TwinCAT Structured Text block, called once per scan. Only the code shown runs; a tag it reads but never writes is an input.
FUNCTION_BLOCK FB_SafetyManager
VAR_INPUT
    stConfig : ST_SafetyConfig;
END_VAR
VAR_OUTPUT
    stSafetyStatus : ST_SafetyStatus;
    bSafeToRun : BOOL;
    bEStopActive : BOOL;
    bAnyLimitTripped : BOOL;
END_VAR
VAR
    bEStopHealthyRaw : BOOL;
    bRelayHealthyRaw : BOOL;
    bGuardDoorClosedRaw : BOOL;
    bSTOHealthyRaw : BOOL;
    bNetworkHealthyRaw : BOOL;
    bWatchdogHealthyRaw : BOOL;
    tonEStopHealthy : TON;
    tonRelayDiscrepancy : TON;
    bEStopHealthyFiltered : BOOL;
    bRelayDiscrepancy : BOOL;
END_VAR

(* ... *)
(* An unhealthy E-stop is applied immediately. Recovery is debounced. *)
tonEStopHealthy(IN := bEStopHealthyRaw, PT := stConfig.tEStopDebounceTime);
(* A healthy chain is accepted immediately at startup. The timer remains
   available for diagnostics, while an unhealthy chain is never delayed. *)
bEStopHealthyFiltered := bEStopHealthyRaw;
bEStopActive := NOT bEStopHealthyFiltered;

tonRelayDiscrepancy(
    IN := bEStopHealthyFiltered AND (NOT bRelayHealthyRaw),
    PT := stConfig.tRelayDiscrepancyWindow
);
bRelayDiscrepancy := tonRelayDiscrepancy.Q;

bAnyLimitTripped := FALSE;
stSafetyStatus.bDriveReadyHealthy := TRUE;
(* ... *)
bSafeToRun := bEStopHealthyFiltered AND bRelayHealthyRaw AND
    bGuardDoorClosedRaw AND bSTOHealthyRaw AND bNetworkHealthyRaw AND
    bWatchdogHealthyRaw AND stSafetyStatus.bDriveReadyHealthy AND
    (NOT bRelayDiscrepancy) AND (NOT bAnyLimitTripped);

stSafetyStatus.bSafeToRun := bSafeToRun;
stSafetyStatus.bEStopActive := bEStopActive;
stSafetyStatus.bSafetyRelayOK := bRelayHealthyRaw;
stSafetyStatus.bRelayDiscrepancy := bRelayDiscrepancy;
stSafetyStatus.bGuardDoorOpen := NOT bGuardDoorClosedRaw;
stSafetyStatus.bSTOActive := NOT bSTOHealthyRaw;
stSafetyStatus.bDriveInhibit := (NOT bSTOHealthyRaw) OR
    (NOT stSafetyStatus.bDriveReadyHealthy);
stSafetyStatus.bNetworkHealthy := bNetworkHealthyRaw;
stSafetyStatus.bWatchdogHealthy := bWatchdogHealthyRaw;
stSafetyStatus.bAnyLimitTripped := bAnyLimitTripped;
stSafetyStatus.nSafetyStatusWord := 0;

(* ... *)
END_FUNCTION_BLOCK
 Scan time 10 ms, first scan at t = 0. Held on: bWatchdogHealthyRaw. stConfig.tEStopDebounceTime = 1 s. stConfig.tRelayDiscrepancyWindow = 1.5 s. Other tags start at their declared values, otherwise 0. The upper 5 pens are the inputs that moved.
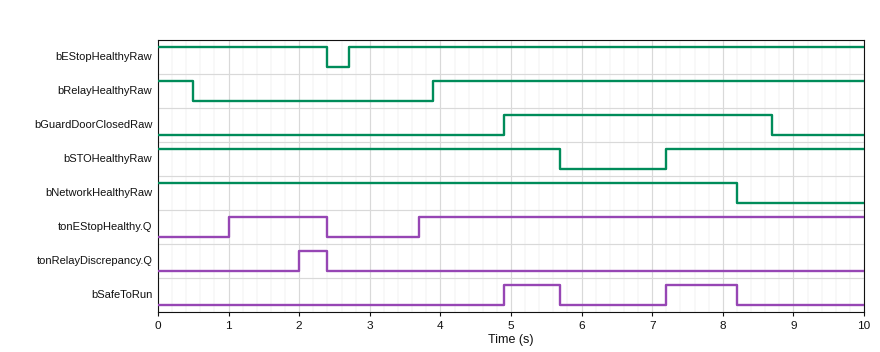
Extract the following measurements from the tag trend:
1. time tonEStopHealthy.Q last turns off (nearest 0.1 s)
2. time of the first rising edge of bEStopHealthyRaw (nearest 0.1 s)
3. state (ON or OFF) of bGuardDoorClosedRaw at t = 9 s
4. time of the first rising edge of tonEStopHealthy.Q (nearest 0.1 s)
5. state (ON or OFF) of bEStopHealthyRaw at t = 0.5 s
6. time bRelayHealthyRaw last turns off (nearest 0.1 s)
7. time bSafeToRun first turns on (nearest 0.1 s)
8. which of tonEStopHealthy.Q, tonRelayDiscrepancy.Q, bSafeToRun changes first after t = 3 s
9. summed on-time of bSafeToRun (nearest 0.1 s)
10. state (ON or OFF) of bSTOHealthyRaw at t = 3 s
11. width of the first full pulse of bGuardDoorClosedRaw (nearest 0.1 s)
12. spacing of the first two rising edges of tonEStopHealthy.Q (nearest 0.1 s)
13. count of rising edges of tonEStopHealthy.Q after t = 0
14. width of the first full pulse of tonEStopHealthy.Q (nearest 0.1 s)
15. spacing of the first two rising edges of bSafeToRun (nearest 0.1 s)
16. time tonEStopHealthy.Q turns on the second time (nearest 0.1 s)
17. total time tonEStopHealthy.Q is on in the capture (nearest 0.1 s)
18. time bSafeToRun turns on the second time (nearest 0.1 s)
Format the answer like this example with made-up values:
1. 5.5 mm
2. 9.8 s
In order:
1. 2.4 s
2. 2.7 s
3. OFF
4. 1.0 s
5. ON
6. 0.5 s
7. 4.9 s
8. tonEStopHealthy.Q
9. 1.8 s
10. ON
11. 3.8 s
12. 2.7 s
13. 2
14. 1.4 s
15. 2.3 s
16. 3.7 s
17. 7.7 s
18. 7.2 s
